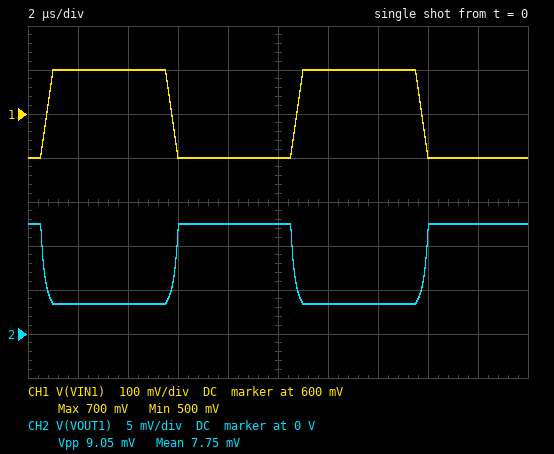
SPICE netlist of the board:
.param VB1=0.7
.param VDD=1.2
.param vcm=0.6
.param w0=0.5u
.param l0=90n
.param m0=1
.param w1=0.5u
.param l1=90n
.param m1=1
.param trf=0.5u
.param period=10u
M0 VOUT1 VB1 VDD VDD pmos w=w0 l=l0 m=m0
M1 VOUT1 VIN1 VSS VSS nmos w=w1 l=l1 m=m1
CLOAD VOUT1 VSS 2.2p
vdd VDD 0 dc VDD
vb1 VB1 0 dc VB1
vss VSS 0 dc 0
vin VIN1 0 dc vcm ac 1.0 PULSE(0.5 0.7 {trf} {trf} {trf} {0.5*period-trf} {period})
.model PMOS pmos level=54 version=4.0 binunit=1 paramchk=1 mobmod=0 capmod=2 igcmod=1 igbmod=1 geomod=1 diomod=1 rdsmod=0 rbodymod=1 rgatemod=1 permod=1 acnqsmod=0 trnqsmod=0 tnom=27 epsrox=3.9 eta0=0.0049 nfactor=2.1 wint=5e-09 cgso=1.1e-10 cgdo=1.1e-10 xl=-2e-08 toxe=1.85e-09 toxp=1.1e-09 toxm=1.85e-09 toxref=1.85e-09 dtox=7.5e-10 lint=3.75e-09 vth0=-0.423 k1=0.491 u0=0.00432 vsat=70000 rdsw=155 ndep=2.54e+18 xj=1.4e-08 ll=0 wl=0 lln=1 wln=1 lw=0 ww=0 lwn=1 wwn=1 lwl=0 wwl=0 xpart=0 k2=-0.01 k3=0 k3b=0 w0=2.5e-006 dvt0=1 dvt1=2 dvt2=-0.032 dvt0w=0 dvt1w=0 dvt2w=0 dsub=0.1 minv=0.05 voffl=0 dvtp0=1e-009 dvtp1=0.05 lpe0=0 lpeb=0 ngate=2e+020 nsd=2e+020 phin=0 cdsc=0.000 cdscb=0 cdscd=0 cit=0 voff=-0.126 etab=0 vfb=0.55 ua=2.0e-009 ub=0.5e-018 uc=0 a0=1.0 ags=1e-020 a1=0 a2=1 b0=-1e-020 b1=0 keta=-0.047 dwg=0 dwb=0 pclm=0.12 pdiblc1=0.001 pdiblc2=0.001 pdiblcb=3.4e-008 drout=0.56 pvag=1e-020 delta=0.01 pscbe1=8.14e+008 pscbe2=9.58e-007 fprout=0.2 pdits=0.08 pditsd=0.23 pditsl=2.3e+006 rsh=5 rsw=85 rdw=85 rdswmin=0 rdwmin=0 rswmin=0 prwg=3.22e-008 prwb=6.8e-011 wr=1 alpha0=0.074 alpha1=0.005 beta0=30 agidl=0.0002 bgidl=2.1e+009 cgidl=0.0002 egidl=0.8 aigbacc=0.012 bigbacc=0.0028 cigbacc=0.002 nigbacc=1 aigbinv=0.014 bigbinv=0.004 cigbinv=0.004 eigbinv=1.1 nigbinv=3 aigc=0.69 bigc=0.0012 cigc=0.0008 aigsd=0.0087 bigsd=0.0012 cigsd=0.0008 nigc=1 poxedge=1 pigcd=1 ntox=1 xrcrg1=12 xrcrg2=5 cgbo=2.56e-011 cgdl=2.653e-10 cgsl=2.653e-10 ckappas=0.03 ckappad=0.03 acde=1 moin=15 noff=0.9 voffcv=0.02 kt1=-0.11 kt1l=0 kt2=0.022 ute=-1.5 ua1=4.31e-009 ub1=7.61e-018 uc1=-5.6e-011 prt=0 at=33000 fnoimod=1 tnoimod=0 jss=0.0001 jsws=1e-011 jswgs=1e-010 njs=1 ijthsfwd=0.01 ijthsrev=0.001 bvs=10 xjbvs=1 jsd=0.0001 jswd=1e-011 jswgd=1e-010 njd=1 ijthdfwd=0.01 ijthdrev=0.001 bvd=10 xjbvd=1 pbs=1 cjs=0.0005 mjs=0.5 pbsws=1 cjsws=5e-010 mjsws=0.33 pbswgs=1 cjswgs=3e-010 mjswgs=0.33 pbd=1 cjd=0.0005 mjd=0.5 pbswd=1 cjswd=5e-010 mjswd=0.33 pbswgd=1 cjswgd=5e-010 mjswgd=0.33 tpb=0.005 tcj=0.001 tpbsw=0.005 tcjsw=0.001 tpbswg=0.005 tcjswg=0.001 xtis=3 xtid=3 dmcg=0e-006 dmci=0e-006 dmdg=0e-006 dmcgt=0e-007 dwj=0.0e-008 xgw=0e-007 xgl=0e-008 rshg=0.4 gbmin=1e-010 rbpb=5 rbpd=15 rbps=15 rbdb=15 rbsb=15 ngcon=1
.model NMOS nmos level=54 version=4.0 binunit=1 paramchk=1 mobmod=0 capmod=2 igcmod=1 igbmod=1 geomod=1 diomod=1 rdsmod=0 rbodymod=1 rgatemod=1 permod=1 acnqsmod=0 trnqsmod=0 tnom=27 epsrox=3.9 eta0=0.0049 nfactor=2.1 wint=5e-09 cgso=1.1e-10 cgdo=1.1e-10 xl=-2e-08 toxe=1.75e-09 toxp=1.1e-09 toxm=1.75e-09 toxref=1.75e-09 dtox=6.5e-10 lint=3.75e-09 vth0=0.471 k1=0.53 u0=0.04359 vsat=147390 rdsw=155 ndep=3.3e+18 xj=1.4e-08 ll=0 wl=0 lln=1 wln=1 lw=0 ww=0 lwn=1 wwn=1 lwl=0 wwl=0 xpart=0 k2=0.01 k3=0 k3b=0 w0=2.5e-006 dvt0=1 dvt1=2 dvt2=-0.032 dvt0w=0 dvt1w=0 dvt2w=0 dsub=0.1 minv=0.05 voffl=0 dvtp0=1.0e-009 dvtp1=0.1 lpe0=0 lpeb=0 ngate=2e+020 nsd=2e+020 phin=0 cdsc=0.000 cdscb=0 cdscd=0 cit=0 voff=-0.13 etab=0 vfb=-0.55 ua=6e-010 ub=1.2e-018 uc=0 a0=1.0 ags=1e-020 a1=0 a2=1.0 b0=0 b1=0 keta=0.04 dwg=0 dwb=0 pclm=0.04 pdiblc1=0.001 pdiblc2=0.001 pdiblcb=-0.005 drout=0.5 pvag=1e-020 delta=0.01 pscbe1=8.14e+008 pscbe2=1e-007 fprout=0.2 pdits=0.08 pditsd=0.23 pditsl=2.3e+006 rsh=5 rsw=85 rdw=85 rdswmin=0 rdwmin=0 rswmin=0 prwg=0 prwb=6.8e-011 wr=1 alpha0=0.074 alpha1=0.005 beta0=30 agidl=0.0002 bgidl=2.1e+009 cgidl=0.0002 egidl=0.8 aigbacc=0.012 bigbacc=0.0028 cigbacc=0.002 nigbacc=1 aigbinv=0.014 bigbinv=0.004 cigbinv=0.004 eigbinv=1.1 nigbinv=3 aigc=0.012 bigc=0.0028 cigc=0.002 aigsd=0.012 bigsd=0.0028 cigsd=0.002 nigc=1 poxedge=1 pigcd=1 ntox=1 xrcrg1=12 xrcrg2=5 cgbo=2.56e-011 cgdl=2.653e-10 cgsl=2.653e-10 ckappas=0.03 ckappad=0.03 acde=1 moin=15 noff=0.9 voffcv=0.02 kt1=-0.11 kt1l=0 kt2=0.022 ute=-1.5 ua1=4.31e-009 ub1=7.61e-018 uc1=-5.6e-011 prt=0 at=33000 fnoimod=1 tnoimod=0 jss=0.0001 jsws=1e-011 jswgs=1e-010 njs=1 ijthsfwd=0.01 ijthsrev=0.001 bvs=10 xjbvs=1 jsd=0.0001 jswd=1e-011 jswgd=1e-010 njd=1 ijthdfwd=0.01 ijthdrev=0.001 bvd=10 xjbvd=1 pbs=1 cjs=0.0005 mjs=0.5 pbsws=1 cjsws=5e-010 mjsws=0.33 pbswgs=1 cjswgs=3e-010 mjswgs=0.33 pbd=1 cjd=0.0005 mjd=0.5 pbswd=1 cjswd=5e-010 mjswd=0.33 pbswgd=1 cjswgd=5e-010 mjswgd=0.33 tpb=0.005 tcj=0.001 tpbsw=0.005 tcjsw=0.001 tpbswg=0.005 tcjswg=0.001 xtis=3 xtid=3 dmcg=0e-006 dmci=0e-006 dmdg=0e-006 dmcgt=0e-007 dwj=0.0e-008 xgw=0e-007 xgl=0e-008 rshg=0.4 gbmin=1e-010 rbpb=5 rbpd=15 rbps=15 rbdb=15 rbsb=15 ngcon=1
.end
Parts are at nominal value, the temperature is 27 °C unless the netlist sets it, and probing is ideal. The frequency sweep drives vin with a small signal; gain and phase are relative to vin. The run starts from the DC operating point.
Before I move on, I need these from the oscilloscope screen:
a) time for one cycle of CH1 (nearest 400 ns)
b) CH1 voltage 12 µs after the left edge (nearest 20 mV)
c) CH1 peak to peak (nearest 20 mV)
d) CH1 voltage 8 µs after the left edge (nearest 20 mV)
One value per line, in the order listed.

10.0 µs
700 mV
200 mV
500 mV
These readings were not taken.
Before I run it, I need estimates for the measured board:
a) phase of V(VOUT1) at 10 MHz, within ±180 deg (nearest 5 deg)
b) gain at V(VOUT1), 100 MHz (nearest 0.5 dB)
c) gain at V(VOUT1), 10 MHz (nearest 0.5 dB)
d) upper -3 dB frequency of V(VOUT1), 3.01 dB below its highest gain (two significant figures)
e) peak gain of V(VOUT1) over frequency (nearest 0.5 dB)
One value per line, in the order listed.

165 deg
-40.0 dB
-30.5 dB
34 MHz
-30.0 dB
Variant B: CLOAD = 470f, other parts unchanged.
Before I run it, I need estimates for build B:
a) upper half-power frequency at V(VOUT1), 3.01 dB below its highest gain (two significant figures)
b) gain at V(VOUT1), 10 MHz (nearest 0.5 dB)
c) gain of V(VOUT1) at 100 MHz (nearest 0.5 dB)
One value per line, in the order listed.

160 MHz
-30.0 dB
-31.5 dB
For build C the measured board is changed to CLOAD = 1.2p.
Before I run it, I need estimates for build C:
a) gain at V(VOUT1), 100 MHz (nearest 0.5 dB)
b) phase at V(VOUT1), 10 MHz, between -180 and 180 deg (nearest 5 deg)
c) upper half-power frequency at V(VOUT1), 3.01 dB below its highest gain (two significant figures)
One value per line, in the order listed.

-35.5 dB
170 deg
62 MHz
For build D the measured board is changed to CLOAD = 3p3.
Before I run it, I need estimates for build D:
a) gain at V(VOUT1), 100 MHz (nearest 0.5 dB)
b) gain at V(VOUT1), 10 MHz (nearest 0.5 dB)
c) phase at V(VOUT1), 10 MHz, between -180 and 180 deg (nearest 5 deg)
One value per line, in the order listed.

-43.5 dB
-31.0 dB
155 deg
